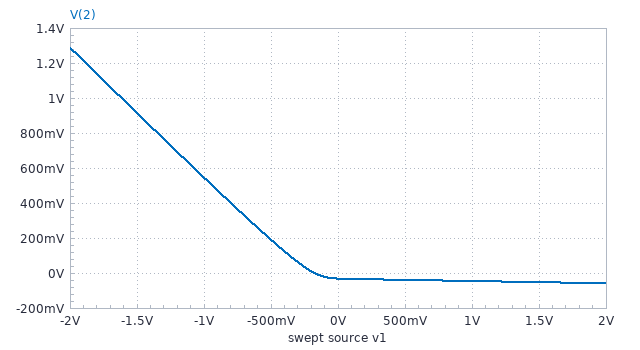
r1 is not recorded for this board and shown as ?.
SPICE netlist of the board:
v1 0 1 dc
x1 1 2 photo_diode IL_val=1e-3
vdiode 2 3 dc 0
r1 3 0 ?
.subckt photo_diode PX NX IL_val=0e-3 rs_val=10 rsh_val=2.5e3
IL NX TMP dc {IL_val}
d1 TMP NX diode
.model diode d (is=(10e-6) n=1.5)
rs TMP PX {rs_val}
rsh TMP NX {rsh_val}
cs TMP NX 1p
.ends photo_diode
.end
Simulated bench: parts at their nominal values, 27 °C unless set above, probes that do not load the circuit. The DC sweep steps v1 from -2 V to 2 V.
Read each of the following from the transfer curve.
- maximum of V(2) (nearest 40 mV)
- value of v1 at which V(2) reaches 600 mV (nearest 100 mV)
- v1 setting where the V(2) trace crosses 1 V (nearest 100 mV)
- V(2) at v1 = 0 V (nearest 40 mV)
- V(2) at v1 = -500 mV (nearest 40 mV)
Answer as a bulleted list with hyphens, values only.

- 1.28 V
- -1.1 V
- -1.6 V
- -40 mV
- 200 mV
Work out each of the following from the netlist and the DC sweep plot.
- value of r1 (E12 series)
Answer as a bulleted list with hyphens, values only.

- 33 Ω
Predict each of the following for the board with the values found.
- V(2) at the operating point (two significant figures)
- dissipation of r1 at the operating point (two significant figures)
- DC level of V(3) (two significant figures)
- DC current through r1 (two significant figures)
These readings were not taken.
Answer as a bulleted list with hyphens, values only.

- -32 mV
- 31 µW
- -32 mV
- 960 µA
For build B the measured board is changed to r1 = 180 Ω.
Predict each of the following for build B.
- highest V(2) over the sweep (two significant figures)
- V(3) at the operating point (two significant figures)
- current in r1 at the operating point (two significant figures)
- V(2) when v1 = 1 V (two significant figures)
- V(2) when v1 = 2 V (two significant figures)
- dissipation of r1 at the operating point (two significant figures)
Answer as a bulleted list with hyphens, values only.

- 1.6 V
- -120 mV
- 680 µA
- -240 mV
- -300 mV
- 83 µW
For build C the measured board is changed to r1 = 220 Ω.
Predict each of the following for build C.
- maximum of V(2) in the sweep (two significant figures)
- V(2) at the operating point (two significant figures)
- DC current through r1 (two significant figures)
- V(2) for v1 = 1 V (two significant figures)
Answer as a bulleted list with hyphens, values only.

- 1.7 V
- -130 mV
- 600 µA
- -280 mV
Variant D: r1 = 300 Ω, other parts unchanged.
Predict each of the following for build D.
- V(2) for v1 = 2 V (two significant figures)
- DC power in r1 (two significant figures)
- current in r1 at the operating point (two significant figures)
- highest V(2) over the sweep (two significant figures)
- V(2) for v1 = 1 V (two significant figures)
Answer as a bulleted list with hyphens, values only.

- -480 mV
- 70 µW
- 480 µA
- 1.7 V
- -380 mV
